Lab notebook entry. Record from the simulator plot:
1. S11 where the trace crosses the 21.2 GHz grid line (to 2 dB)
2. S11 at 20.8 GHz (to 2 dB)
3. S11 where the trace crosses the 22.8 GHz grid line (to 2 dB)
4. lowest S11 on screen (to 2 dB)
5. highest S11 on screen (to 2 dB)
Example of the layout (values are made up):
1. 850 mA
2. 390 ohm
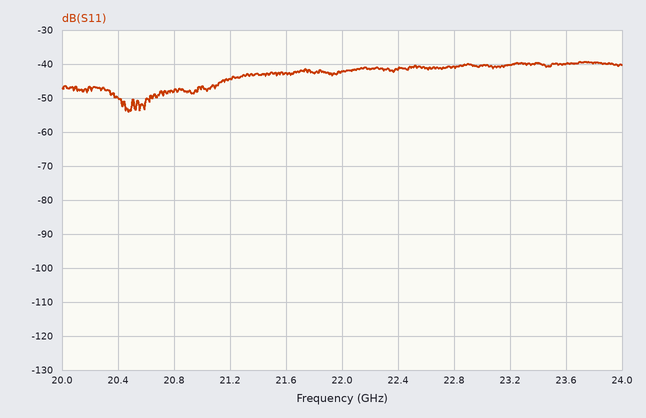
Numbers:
1. -44 dB
2. -48 dB
3. -40 dB
4. -54 dB
5. -40 dB
